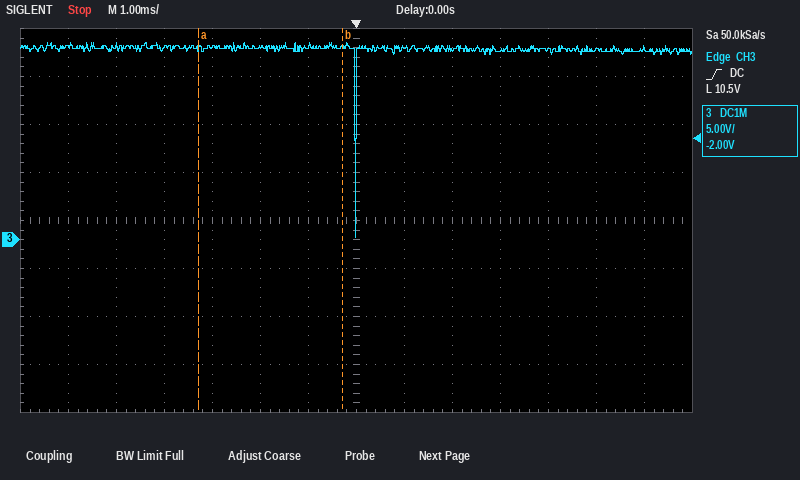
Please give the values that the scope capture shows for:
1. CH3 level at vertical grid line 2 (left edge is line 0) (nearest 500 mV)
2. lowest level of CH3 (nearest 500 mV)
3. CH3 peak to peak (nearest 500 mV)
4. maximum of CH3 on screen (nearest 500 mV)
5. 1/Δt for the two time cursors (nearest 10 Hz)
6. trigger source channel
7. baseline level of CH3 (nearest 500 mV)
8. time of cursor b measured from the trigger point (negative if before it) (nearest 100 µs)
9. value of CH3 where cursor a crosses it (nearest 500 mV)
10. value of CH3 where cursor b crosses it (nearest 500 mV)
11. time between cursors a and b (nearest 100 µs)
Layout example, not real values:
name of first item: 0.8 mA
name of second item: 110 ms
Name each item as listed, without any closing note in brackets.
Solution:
CH3 level at vertical grid line 2 (left edge is line 0): 20.0 V
lowest level of CH3: 0.0 V
CH3 peak to peak: 20.5 V
maximum of CH3 on screen: 20.5 V
1/Δt for the two time cursors: 330 Hz
trigger source channel: CH3
baseline level of CH3: 20.0 V
time of cursor b measured from the trigger point (negative if before it): -300 µs
value of CH3 where cursor a crosses it: 20.0 V
value of CH3 where cursor b crosses it: 20.0 V
time between cursors a and b: 3.0 ms
